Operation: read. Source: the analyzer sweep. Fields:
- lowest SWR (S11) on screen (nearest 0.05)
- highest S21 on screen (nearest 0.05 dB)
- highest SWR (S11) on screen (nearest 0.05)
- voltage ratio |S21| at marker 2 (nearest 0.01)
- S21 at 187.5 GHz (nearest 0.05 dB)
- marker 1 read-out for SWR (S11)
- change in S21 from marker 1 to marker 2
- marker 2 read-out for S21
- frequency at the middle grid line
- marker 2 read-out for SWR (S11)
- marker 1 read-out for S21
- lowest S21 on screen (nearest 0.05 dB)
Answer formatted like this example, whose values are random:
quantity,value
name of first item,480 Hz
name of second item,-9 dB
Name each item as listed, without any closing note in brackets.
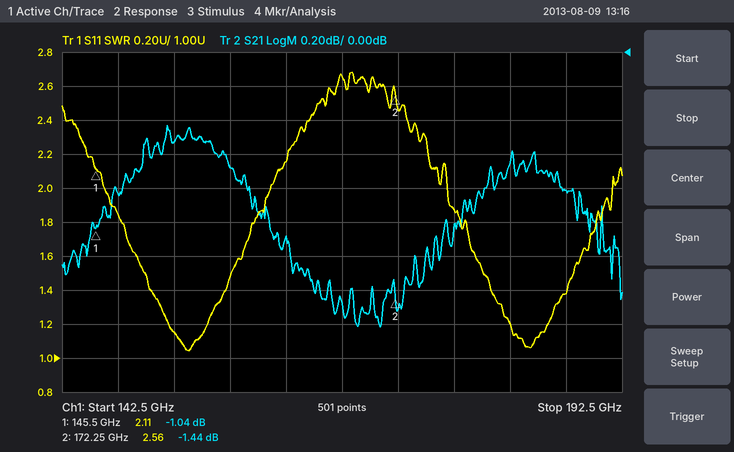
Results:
quantity,value
lowest SWR (S11) on screen,1.05
highest S21 on screen,-0.45 dB
highest SWR (S11) on screen,2.70
voltage ratio |S21| at marker 2,0.85
S21 at 187.5 GHz,-0.80 dB
marker 1 read-out for SWR,2.11
change in S21 from marker 1 to marker 2,-0.40 dB
marker 2 read-out for S21,-1.44 dB
frequency at the middle grid line,167.5 GHz
marker 2 read-out for SWR,2.56
marker 1 read-out for S21,-1.04 dB
lowest S21 on screen,-1.60 dB
